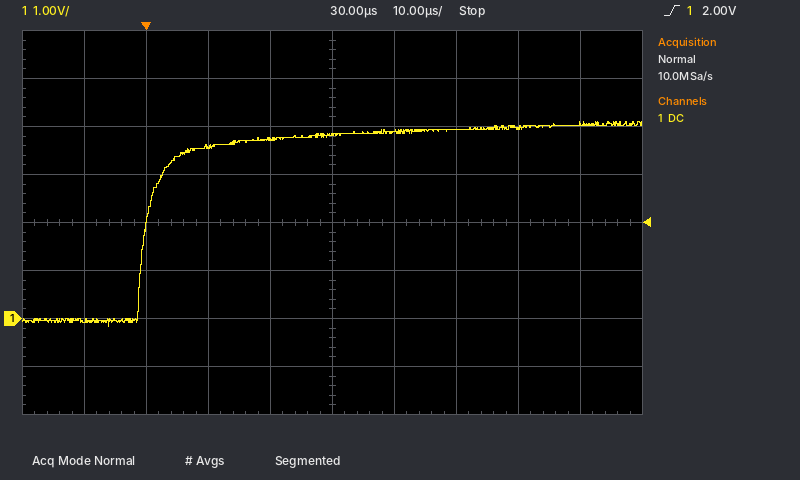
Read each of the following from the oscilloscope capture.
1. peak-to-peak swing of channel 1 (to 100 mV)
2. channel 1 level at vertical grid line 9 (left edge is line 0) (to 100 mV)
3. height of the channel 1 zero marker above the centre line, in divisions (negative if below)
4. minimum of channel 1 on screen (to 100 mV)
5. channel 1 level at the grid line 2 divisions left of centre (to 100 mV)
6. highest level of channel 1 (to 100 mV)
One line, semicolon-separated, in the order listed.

4.3 V; 4.1 V; -2.0 div; -200 mV; 3.6 V; 4.1 V
